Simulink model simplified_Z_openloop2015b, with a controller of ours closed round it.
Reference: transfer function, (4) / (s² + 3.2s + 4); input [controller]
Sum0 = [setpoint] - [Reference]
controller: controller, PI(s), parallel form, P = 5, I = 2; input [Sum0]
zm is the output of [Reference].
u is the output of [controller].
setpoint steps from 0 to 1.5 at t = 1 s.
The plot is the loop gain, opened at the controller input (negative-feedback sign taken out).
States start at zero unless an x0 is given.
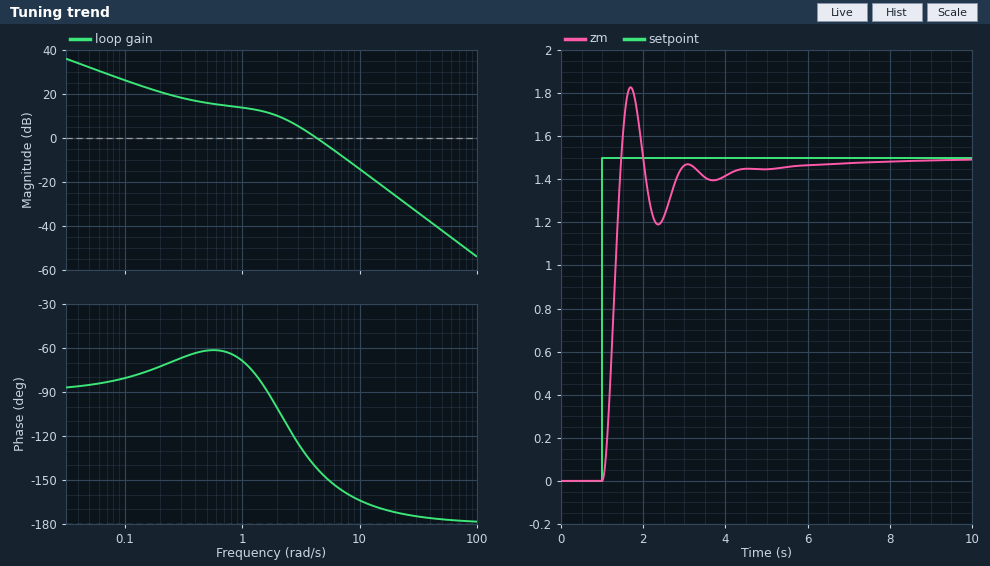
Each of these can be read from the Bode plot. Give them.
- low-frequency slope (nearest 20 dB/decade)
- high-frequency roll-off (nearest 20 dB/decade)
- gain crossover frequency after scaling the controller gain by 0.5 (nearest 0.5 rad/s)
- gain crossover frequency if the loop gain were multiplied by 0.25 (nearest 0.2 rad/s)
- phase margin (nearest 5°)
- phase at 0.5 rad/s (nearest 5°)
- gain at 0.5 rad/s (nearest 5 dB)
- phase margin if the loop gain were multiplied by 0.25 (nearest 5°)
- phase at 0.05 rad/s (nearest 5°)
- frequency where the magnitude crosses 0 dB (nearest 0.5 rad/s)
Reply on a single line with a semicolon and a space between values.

-20 dB/decade; -40 dB/decade; 3.0 rad/s; 1.6 rad/s; 40°; -60°; 15 dB; 95°; -85°; 4.5 rad/s
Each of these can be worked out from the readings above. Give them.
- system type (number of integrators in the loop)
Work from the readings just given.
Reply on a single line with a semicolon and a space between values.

1
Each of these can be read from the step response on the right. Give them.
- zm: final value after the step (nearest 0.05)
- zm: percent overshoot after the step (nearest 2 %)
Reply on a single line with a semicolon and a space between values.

1.50; 22 %
